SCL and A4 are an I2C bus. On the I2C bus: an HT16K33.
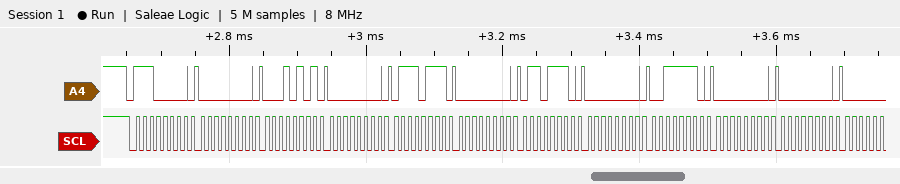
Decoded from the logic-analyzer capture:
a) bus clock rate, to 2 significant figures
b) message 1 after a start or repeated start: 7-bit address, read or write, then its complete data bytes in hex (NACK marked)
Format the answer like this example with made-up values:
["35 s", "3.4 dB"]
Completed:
["100 kHz", "0x70 write: 00 15 00 77 00 6E 00 3E 00 00"]
